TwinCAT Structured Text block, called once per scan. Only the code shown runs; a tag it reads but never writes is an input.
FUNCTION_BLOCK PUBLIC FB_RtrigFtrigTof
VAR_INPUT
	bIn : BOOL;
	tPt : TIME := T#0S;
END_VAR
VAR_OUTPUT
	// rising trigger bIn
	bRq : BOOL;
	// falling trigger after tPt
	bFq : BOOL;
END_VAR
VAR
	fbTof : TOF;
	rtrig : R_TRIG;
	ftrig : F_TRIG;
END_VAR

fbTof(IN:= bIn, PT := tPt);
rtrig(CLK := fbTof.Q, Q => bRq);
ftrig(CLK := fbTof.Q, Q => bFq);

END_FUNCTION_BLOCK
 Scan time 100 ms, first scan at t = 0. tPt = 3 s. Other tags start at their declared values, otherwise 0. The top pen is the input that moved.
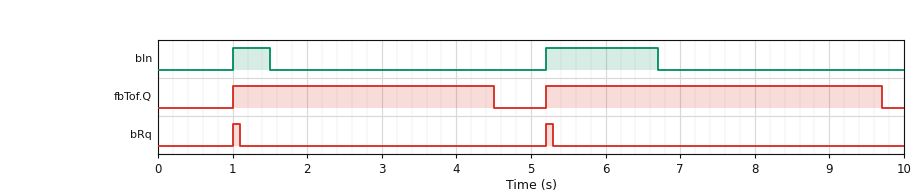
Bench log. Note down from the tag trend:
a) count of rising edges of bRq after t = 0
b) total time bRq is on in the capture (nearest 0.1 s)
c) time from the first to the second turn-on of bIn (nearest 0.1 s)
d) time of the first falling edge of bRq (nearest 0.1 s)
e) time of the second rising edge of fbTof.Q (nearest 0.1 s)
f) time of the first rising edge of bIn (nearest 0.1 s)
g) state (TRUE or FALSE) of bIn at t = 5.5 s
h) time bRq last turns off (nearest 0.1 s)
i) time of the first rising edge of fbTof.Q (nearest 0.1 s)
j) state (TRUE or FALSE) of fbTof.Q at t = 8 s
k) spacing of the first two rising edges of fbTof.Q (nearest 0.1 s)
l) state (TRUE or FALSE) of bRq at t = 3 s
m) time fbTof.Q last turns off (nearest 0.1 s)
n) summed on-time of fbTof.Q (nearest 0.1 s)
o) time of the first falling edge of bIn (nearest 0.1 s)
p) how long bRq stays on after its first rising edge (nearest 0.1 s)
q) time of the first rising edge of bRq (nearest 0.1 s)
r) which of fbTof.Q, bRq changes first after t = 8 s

2
0.2 s
4.2 s
1.1 s
5.2 s
1.0 s
TRUE
5.3 s
1.0 s
TRUE
4.2 s
FALSE
9.7 s
8.0 s
1.5 s
0.1 s
1.0 s
fbTof.Q
